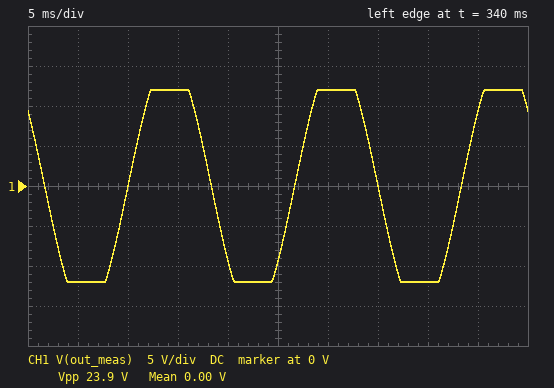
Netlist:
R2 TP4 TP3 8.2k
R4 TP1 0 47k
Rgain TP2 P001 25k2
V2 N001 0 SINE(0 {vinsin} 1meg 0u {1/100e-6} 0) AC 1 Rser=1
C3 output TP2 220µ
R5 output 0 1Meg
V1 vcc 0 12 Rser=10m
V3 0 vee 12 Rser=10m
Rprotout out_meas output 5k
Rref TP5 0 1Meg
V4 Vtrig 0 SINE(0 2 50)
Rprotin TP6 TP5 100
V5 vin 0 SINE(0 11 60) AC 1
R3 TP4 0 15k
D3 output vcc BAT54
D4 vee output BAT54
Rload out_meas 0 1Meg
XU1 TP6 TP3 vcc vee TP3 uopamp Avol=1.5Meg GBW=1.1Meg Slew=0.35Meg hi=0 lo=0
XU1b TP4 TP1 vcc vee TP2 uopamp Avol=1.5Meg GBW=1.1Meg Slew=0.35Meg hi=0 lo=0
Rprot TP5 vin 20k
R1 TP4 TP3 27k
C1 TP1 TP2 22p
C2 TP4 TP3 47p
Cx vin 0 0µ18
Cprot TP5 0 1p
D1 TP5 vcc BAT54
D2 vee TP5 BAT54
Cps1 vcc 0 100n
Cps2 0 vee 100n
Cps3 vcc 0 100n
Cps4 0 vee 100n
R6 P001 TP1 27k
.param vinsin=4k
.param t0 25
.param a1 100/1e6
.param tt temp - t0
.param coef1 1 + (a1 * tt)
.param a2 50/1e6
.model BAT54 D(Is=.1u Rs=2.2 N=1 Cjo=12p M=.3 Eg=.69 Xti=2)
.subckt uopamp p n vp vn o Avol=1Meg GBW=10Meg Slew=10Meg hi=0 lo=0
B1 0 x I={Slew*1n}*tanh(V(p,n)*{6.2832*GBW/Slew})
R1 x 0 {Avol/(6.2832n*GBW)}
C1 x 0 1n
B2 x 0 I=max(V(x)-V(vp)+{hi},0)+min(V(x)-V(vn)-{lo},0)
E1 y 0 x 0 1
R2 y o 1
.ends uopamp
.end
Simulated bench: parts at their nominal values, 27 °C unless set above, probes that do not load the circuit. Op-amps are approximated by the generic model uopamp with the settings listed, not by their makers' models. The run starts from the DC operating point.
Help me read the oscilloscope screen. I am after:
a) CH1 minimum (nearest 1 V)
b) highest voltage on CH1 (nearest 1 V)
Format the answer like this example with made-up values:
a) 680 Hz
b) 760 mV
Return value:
a) -12 V
b) 12 V
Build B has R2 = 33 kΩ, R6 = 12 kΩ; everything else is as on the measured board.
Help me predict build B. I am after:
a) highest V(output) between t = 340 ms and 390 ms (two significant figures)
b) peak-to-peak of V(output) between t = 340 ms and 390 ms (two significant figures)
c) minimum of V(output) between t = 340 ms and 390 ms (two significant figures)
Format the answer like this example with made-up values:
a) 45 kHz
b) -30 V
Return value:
a) 9.7 V
b) 19 V
c) -9.7 V
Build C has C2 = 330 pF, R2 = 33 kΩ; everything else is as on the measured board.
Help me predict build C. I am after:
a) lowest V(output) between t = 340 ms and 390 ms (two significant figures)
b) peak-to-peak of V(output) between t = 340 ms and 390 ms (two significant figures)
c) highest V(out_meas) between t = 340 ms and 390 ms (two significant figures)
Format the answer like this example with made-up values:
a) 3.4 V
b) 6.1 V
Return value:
a) -11 V
b) 23 V
c) 11 V
